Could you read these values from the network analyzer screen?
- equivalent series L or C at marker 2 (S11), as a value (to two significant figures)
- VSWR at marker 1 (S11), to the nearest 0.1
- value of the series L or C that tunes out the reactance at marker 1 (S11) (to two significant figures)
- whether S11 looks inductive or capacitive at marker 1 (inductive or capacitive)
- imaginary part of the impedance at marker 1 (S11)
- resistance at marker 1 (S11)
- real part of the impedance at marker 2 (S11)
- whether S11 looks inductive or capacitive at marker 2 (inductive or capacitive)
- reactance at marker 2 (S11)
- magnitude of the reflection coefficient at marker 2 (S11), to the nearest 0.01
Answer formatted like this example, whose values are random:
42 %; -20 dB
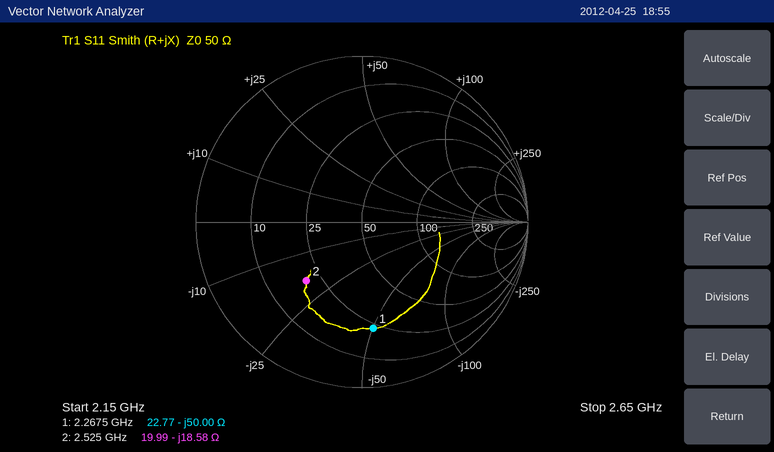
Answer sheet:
3.4 pF; 4.6; 3.5 nH; capacitive; -50.00 Ω; 22.77 Ω; 19.99 Ω; capacitive; -18.58 Ω; 0.49
